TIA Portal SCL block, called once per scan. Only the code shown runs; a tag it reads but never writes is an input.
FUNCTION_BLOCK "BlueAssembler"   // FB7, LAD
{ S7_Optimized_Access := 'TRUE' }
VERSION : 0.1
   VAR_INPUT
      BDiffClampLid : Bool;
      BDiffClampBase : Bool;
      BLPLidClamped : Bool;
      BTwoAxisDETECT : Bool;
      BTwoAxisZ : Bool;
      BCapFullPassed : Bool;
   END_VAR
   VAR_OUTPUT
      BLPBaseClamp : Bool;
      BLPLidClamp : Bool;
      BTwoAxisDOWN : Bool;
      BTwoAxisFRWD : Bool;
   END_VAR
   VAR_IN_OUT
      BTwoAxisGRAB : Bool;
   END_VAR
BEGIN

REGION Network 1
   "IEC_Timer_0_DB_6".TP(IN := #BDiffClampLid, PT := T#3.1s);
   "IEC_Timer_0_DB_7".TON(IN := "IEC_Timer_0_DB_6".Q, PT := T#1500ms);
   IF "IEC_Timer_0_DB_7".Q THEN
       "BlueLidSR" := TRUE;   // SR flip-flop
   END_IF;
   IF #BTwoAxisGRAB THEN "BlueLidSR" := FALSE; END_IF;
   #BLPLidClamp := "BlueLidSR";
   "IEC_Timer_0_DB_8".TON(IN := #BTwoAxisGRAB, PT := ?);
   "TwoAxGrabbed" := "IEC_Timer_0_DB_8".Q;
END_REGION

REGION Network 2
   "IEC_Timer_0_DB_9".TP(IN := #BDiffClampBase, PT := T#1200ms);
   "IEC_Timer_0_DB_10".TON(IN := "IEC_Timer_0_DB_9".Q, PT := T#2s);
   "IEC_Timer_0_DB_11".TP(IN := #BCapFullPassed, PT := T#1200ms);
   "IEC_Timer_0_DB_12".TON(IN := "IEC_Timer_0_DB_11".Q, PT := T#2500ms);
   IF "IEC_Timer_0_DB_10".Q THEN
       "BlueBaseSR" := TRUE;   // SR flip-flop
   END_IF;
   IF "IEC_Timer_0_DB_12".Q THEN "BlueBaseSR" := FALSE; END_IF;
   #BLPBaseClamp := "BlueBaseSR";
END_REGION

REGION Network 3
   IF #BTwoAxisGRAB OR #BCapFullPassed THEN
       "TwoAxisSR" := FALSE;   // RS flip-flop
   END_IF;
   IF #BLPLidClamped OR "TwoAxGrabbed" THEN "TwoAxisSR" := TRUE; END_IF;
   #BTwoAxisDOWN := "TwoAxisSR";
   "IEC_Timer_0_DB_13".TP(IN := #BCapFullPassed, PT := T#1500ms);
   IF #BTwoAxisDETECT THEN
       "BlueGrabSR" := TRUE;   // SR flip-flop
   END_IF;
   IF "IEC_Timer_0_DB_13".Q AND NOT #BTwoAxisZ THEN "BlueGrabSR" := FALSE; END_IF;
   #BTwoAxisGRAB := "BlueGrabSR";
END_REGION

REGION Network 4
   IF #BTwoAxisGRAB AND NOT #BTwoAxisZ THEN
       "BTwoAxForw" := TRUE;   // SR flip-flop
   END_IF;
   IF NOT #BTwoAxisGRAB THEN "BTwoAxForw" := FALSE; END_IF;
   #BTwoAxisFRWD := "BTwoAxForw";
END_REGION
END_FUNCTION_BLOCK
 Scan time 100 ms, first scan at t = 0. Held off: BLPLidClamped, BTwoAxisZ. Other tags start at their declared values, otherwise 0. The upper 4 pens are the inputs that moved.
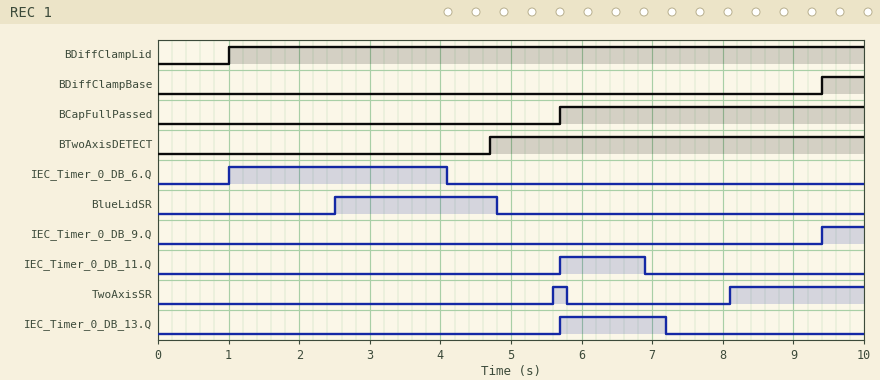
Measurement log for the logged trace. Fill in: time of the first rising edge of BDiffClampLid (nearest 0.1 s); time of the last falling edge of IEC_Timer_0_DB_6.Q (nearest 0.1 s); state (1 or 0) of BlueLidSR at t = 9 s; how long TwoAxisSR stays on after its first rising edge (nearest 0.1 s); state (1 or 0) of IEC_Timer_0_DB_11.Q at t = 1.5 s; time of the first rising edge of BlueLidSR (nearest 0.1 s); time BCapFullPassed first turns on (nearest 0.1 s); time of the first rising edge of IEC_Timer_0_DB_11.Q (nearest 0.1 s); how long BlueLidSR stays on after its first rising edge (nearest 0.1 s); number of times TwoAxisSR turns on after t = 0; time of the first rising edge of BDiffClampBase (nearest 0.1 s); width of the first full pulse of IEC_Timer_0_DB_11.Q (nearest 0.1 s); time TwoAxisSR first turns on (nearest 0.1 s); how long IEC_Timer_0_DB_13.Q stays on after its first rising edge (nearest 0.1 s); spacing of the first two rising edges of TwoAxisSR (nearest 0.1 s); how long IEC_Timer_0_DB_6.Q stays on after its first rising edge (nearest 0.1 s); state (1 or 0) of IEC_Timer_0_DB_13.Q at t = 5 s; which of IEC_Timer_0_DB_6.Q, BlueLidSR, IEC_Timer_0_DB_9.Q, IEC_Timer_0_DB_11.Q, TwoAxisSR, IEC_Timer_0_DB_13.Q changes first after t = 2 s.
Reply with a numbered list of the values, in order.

1. 1.0 s
2. 4.1 s
3. 0
4. 0.2 s
5. 0
6. 2.5 s
7. 5.7 s
8. 5.7 s
9. 2.3 s
10. 2
11. 9.4 s
12. 1.2 s
13. 5.6 s
14. 1.5 s
15. 2.5 s
16. 3.1 s
17. 0
18. BlueLidSR
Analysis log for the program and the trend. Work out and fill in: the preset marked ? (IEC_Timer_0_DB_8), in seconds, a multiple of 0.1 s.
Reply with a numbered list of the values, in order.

1. 0.8 s
